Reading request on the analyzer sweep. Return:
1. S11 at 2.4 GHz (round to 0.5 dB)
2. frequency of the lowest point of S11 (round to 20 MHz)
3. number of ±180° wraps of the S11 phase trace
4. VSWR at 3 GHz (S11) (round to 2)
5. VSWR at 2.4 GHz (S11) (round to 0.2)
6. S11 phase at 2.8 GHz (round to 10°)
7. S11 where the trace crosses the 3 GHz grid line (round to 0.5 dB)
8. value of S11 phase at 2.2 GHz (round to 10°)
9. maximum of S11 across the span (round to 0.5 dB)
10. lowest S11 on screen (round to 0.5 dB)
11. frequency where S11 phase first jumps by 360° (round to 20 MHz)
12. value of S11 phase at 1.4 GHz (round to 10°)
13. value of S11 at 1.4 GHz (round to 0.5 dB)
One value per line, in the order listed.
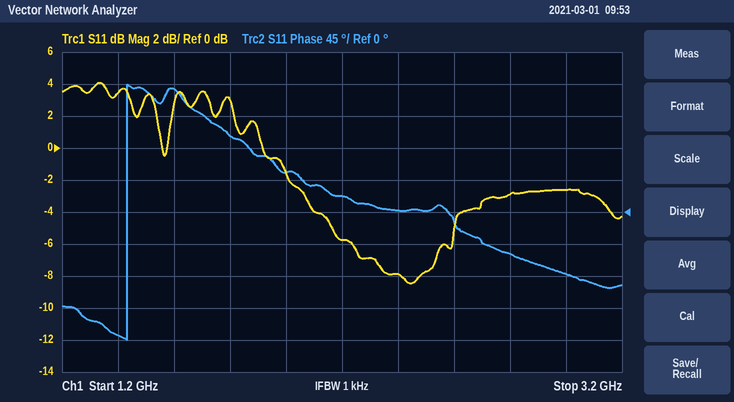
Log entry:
-8.0 dB
2.44 GHz
1
6
2.4
-60°
-2.5 dB
20°
4.0 dB
-8.5 dB
1.44 GHz
-170°
3.5 dB
